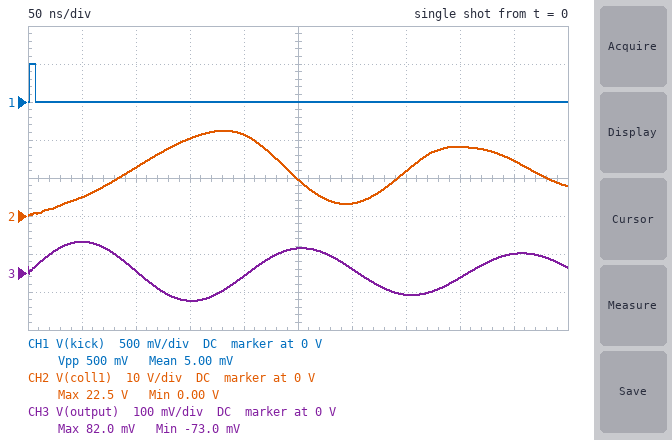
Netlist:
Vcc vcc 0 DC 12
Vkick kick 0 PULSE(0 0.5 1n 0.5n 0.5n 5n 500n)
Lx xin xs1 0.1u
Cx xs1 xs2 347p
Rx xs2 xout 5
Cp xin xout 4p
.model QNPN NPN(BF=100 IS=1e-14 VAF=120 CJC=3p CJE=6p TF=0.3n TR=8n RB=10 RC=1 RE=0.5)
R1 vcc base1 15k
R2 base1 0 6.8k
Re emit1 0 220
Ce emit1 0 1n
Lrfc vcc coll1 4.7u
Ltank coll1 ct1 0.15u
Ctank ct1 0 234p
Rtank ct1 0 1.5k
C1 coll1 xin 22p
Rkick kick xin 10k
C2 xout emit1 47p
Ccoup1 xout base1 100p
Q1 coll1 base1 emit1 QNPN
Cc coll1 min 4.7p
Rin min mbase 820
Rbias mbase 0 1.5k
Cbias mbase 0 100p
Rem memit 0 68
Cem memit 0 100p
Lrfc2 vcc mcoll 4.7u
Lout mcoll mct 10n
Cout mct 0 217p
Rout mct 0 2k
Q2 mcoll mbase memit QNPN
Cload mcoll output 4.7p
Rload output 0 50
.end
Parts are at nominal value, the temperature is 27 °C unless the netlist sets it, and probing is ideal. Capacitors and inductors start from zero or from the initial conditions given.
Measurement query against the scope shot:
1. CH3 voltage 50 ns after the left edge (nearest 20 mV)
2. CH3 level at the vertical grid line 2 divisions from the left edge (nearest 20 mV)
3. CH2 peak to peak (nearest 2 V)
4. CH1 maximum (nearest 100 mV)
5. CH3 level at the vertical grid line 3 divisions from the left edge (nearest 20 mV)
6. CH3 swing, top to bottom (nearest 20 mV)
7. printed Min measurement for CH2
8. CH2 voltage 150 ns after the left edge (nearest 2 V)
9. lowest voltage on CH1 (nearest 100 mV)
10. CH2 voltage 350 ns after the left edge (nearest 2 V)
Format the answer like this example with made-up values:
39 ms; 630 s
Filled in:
80 mV; 0 V; 22 V; 500 mV; -80 mV; 160 mV; 0.00 V; 20 V; 0 V; 12 V
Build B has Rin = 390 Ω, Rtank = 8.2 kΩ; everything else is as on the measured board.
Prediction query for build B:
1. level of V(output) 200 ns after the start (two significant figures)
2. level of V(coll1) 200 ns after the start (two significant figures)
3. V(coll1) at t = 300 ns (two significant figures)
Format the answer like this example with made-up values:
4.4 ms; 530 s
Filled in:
-7.8 mV; 22 V; 1.5 V
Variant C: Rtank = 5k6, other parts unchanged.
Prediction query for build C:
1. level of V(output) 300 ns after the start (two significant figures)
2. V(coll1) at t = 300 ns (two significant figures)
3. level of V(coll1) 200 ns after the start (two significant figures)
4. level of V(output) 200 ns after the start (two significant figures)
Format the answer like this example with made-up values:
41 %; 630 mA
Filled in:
11 mV; 1.7 V; 22 V; -7.9 mV
